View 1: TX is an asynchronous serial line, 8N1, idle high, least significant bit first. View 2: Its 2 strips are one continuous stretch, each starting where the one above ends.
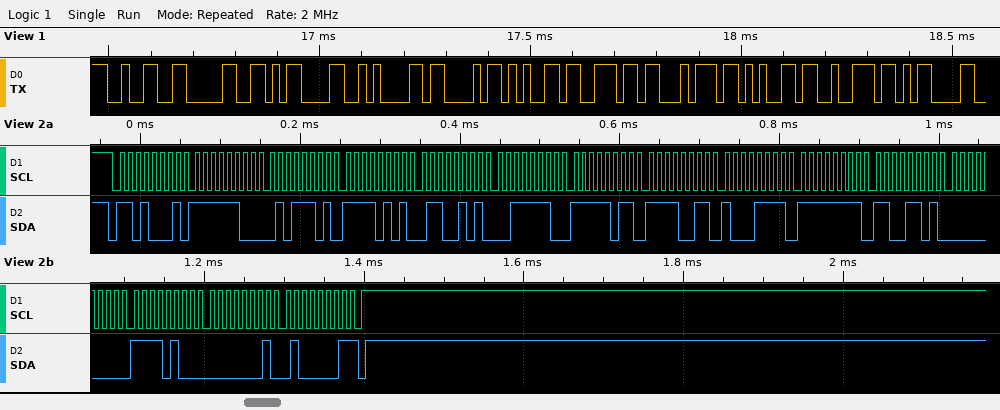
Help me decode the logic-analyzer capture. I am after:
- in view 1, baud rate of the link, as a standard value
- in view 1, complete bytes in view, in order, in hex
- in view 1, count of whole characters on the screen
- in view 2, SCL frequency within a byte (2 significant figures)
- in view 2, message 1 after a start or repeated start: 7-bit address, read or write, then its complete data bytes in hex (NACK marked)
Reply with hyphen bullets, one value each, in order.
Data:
- 57600 baud
- 32 30 0D 0A 43 65 6E 74 65 72 0D
- 11
- 100 kHz
- 0x68 read: FC 5D F5 65 3E FB F3 8F FF CD 00 F4 01 41 NACK
